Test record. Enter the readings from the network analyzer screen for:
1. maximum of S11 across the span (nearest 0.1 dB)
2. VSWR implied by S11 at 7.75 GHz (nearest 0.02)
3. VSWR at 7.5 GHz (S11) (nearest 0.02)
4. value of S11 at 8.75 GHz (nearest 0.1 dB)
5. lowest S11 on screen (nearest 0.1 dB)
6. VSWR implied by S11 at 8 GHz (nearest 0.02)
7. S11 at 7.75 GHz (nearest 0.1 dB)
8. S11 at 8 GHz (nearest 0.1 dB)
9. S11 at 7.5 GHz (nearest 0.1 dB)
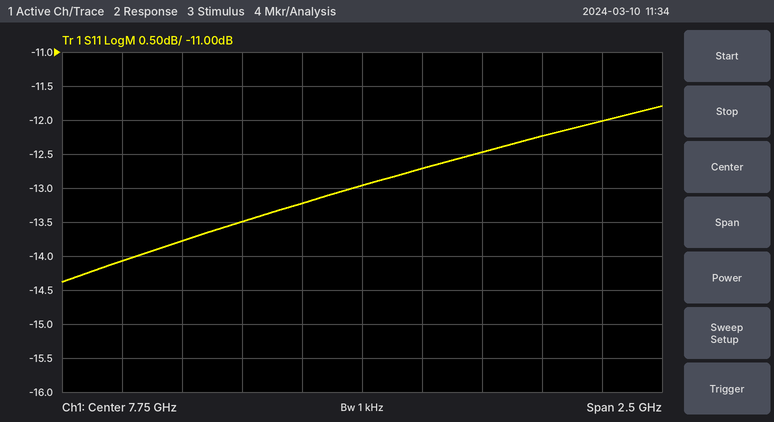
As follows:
-11.8 dB
1.58
1.56
-12.0 dB
-14.4 dB
1.60
-13.0 dB
-12.7 dB
-13.2 dB
